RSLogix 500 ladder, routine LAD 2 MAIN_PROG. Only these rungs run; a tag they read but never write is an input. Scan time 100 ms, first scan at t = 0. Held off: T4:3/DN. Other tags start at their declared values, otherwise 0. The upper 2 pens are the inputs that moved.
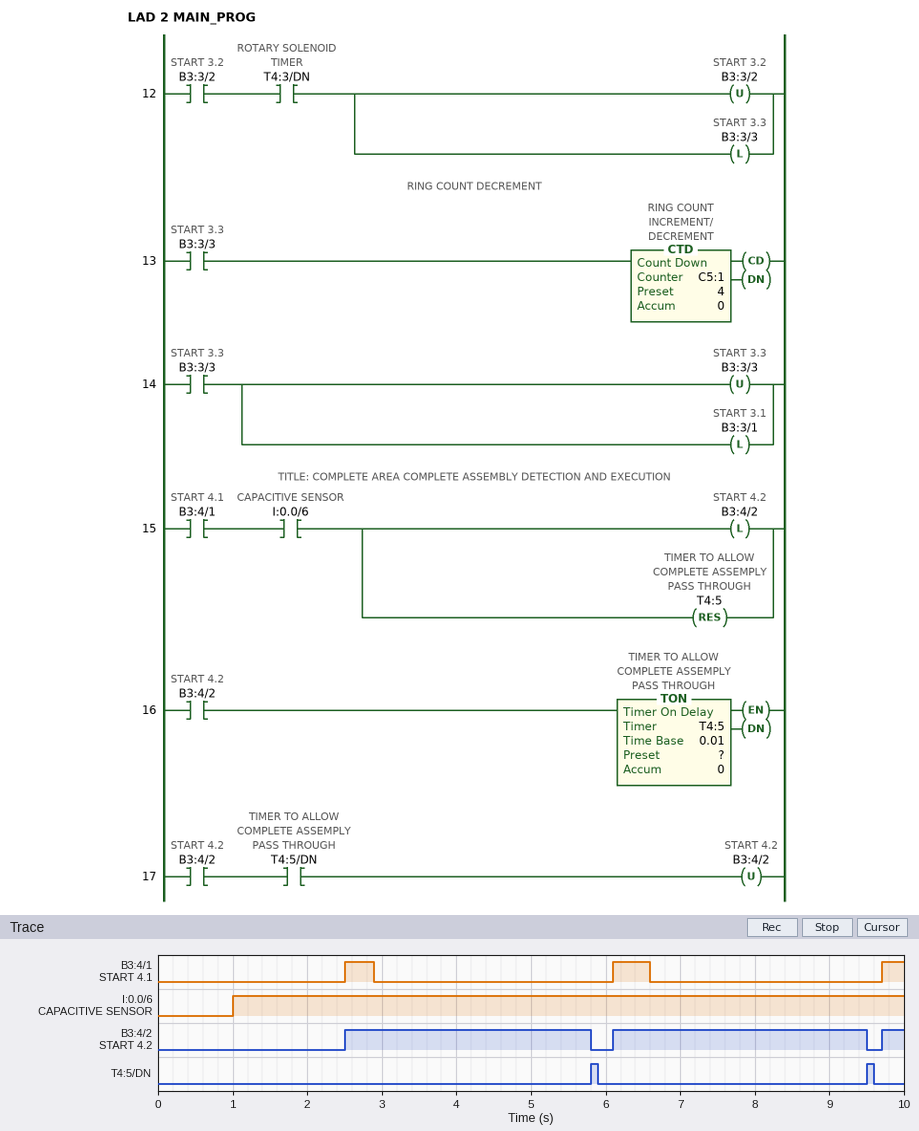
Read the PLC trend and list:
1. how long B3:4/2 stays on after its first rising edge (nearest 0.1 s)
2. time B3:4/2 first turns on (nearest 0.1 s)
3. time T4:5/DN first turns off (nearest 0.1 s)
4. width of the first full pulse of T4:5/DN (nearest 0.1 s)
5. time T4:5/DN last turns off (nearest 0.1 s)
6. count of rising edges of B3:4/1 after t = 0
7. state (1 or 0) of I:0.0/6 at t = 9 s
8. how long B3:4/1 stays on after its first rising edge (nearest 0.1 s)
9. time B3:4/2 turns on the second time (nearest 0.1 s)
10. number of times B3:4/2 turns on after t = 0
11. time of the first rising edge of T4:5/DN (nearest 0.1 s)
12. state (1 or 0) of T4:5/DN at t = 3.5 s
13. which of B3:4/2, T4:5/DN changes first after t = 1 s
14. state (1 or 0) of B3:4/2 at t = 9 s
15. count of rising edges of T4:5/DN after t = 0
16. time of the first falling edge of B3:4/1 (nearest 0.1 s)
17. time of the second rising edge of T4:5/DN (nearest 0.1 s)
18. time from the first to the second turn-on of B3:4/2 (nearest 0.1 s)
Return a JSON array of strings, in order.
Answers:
["3.3 s", "2.5 s", "5.9 s", "0.1 s", "9.6 s", "3", "1", "0.4 s", "6.1 s", "3", "5.8 s", "0", "B3:4/2", "1", "2", "2.9 s", "9.5 s", "3.6 s"]
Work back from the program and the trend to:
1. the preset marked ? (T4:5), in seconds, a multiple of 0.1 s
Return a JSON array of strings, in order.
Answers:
["3.0 s"]
